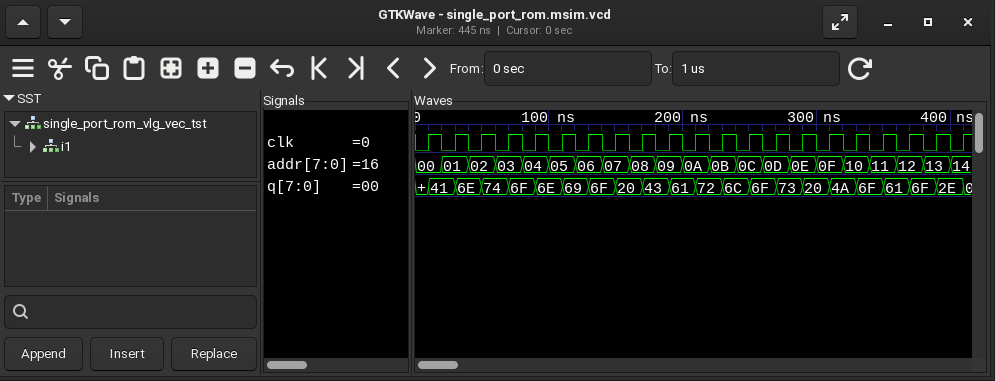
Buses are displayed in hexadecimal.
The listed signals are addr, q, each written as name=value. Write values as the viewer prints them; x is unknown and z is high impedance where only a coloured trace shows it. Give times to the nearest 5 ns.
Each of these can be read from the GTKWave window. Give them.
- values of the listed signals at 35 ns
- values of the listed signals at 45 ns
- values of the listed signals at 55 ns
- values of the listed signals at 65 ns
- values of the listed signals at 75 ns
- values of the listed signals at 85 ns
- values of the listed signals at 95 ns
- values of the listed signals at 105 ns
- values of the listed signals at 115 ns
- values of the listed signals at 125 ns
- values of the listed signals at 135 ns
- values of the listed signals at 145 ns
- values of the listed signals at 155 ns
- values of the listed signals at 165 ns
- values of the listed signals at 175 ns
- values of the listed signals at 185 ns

addr=01, q=6E
addr=02, q=6E
addr=02, q=74
addr=03, q=74
addr=03, q=6F
addr=04, q=6F
addr=04, q=6E
addr=05, q=6E
addr=05, q=69
addr=06, q=69
addr=06, q=6F
addr=07, q=6F
addr=07, q=20
addr=08, q=20
addr=08, q=43
addr=09, q=43
